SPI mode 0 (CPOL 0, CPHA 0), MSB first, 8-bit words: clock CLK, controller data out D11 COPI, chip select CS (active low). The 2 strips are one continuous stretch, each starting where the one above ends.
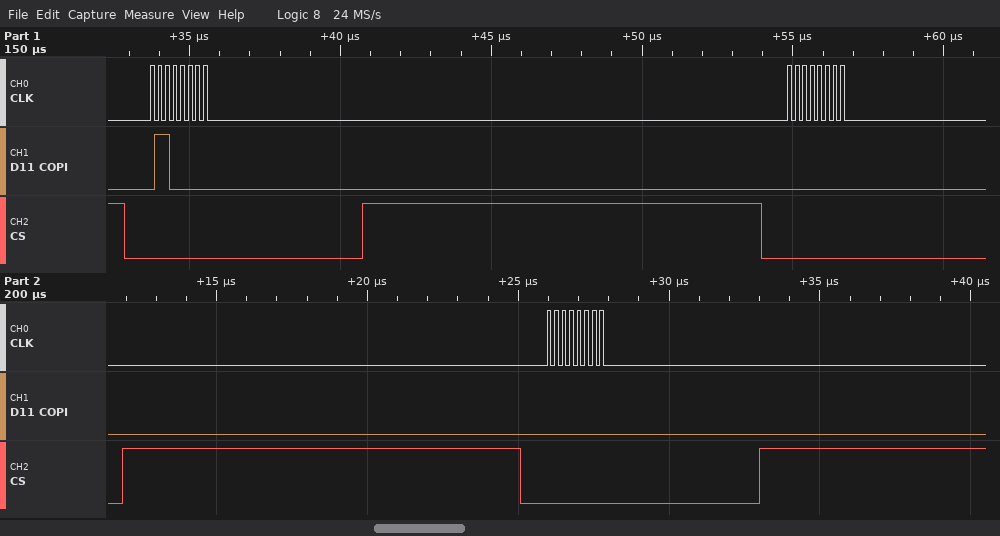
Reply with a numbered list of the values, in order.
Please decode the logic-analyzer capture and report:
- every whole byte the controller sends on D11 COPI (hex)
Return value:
1. 60 00 00
